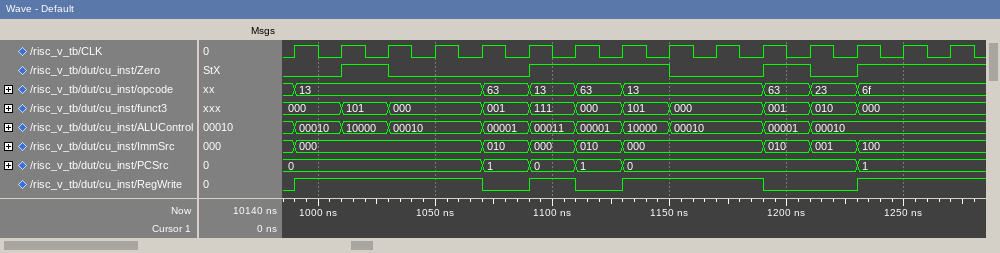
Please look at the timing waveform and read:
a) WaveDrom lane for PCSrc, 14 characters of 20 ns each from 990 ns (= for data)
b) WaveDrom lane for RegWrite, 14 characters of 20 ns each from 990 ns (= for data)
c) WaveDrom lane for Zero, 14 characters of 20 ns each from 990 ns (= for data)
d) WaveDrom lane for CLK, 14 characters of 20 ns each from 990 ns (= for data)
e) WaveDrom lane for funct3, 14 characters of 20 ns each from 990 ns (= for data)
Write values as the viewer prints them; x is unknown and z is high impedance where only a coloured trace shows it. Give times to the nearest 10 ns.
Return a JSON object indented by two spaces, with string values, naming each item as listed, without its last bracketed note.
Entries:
{
  "WaveDrom lane for PCSrc, 14 characters of 20 ns each from 990 ns": "{name: 'PCSrc', wave: '=...====....=.', data: '0 1 0 1 0 1'}",
  "WaveDrom lane for RegWrite, 14 characters of 20 ns each from 990 ns": "{name: 'RegWrite', wave: '1...0101..0.1.'}",
  "WaveDrom lane for Zero, 14 characters of 20 ns each from 990 ns": "{name: 'Zero', wave: '010..1..0.101.'}",
  "WaveDrom lane for CLK, 14 characters of 20 ns each from 990 ns": "{name: 'CLK', wave: 'p.............'}",
  "WaveDrom lane for funct3, 14 characters of 20 ns each from 990 ns": "{name: 'funct3', wave: '===.=====.===.', data: '000 101 000 001 111 000 101 000 001 010 000'}"
}
